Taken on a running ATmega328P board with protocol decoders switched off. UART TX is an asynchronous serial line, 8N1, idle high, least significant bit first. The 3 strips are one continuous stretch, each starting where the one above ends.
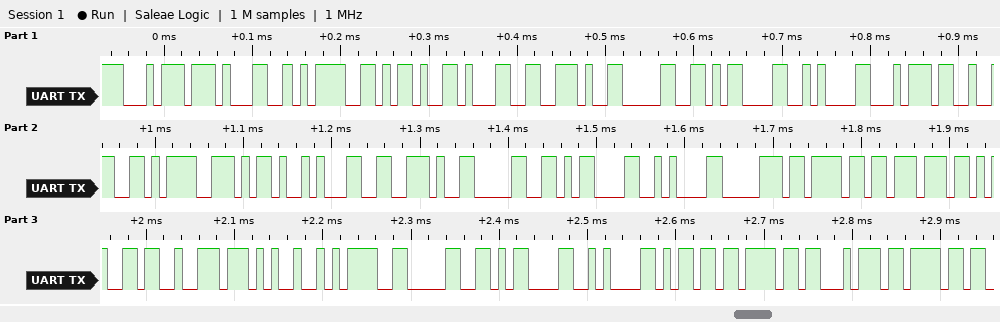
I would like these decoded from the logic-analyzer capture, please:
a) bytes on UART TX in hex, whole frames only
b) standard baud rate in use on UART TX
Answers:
74 31 3D 2D 31 2E 30 0D 0A 74 32 3D 2D 31 2E 30 0D 0A 70 6F 77 65 72 25 3D 30 0D 0A 6D 6F 74 6F
115200 baud
